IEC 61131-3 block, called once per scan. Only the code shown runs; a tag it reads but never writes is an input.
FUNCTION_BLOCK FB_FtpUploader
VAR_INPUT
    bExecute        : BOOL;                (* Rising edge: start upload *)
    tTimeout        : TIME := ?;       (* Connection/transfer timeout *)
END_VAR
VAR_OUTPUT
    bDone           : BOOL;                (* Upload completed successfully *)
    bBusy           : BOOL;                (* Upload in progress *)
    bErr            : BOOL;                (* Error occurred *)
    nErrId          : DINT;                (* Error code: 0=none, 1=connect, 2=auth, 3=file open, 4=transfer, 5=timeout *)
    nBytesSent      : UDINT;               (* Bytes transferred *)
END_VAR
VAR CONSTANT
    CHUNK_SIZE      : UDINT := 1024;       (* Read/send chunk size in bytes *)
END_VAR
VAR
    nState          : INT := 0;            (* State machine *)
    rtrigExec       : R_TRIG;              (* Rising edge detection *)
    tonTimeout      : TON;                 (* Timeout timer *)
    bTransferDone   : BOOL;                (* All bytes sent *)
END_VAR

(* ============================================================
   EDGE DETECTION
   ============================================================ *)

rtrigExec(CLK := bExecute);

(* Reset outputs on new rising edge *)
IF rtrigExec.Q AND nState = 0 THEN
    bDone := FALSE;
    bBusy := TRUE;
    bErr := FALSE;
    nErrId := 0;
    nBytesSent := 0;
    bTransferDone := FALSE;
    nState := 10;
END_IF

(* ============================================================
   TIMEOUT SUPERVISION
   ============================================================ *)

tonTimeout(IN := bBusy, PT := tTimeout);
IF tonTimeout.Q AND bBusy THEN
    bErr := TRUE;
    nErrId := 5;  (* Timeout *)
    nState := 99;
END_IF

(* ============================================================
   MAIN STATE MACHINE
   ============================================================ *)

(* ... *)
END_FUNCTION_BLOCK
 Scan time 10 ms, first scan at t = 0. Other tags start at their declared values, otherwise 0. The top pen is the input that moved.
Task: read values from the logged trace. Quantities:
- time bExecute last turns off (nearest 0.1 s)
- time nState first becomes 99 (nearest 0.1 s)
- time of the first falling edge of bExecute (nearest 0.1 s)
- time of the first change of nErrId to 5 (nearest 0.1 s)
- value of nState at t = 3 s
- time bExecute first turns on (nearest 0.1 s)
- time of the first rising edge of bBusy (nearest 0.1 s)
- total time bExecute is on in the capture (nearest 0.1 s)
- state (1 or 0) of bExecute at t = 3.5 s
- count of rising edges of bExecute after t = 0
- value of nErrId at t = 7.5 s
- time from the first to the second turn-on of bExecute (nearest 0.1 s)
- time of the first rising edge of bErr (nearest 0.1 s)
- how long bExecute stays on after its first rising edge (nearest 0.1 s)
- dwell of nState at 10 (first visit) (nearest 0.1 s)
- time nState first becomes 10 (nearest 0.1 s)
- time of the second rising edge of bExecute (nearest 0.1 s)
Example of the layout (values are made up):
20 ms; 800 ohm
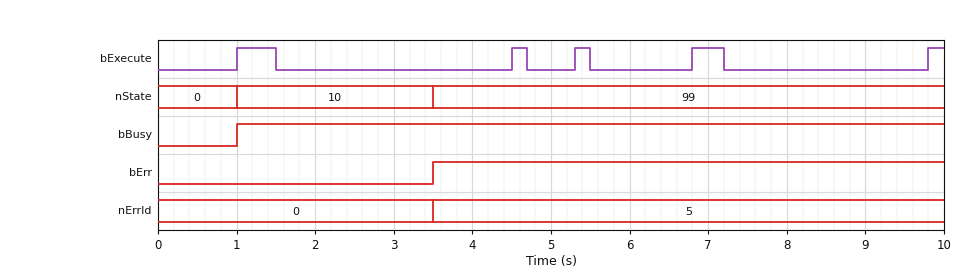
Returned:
7.2 s; 3.5 s; 1.5 s; 3.5 s; 10; 1.0 s; 1.0 s; 1.5 s; 0; 5; 5; 3.5 s; 3.5 s; 0.5 s; 2.5 s; 1.0 s; 4.5 s
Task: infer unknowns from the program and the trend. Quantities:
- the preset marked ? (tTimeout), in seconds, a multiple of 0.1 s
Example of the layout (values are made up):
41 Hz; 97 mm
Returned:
2.5 s
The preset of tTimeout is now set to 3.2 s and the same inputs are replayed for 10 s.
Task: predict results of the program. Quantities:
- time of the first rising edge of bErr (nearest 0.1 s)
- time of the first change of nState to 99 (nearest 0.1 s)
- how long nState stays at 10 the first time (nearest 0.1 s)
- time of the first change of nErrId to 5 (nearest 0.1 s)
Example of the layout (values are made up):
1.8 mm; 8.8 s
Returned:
4.2 s; 4.2 s; 3.2 s; 4.2 s
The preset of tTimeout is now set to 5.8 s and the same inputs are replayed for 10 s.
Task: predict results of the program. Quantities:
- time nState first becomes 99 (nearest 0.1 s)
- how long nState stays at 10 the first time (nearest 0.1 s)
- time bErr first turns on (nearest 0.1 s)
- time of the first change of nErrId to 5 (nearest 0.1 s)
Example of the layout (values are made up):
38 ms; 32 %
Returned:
6.8 s; 5.8 s; 6.8 s; 6.8 s
